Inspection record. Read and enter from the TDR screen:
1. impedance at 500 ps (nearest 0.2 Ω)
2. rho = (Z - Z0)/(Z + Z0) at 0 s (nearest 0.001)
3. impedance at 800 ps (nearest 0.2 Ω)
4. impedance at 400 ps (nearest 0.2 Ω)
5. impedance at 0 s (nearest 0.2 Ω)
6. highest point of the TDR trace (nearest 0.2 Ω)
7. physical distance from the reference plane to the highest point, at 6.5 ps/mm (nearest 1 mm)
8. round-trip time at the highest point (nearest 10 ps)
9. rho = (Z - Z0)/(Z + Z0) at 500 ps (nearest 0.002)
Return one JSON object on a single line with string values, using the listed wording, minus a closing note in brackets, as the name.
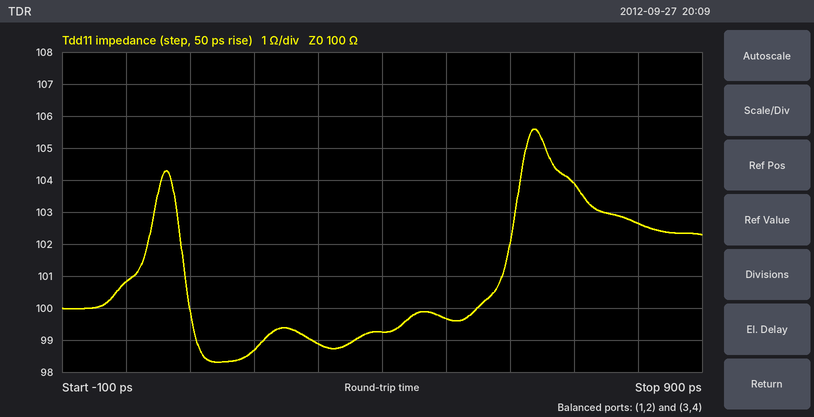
{"impedance at 500 ps": "99.6 Ω", "rho = (Z - Z0)/(Z + Z0) at 0 s": "+0.004", "impedance at 800 ps": "102.6 Ω", "impedance at 400 ps": "99.2 Ω", "impedance at 0 s": "100.8 Ω", "highest point of the TDR trace": "105.6 Ω", "physical distance from the reference plane to the highest point, at 6.5 ps/mm": "49 mm", "round-trip time at the highest point": "640 ps", "rho = (Z - Z0)/(Z + Z0) at 500 ps": "-0.002"}
